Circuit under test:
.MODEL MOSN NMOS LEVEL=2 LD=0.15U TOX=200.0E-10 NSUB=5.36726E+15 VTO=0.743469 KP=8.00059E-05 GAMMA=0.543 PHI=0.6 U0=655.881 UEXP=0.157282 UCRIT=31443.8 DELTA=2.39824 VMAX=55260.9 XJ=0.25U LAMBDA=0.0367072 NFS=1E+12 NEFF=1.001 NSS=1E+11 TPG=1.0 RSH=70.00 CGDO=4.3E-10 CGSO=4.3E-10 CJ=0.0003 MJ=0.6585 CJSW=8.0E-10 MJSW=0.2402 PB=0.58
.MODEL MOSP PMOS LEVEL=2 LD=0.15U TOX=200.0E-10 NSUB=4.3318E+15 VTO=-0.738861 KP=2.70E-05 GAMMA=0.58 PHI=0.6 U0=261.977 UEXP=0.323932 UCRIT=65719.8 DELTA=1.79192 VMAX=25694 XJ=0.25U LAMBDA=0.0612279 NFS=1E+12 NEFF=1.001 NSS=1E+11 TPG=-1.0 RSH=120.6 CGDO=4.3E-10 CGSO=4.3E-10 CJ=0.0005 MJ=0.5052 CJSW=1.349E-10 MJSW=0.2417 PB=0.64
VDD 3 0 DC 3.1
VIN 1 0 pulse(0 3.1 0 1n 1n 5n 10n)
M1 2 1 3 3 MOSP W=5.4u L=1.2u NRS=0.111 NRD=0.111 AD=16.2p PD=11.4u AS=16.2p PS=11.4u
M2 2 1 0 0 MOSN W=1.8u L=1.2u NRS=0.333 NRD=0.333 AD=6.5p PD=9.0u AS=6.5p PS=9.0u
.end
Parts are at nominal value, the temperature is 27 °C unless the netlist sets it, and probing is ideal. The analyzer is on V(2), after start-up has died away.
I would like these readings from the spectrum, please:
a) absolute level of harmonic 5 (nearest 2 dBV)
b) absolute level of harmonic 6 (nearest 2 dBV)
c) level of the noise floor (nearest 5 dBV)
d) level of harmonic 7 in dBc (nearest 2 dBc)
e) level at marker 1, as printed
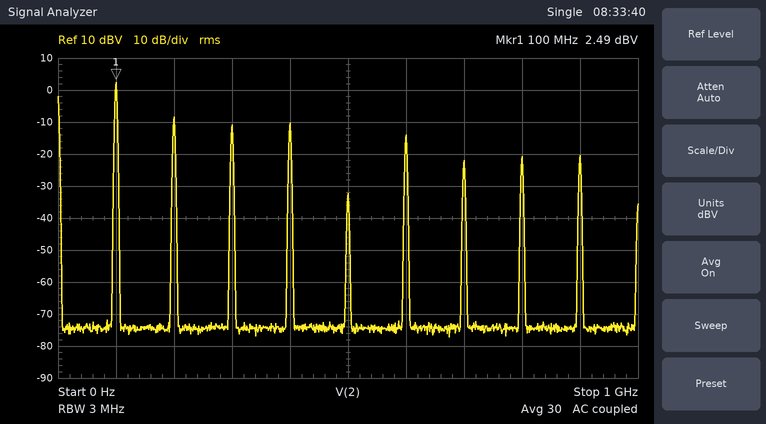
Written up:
-32 dBV
-14 dBV
-75 dBV
-24 dBc
2.49 dBV
